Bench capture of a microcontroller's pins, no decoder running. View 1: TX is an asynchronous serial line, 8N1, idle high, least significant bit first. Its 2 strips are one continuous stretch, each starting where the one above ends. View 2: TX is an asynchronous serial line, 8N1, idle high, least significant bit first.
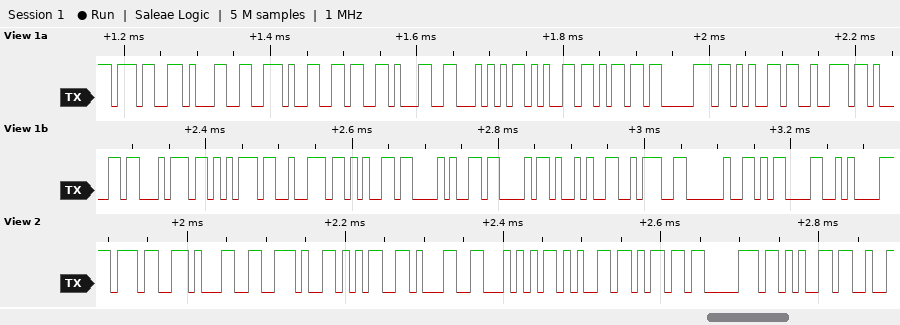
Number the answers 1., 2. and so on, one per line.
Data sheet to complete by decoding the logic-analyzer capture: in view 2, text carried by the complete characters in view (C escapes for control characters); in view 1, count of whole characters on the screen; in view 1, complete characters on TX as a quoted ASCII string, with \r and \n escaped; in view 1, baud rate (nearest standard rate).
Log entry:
1. "71.51Tempe"
2. 23
3. "71.61Temperature(C): \r\n"
4. 115200 baud
